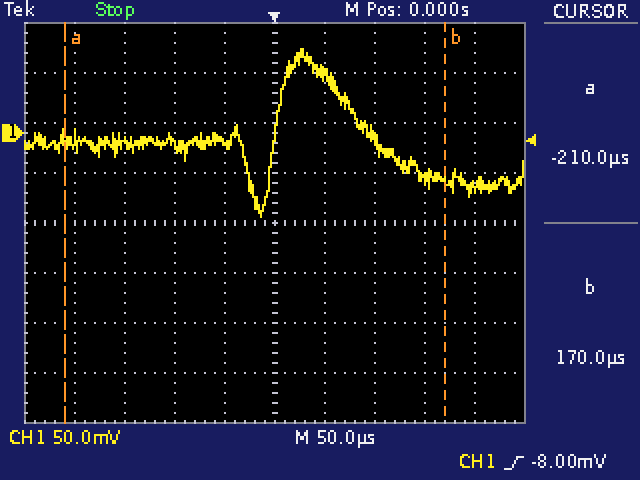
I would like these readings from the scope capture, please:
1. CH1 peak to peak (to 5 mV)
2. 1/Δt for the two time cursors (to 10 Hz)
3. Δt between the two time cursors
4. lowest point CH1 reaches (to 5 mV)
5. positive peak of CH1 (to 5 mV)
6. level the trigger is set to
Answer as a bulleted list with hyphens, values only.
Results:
- 170 mV
- 2.63 kHz
- 380 µs
- -85 mV
- 85 mV
- -8.00 mV
